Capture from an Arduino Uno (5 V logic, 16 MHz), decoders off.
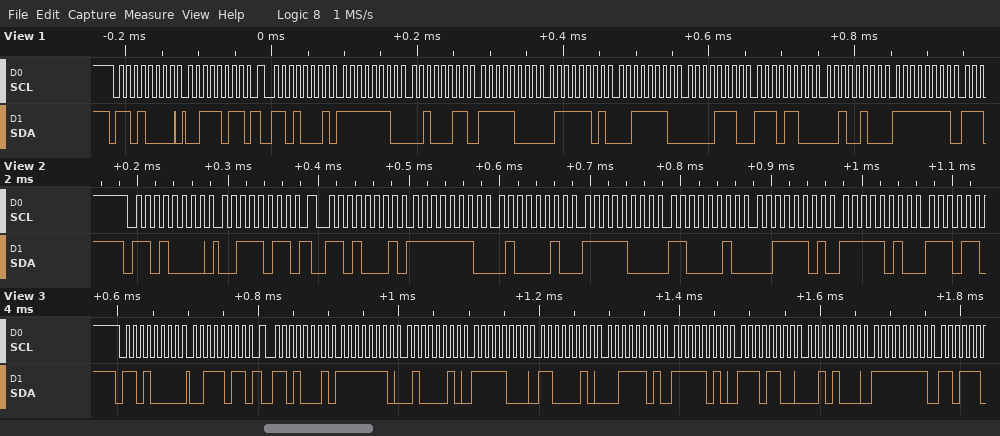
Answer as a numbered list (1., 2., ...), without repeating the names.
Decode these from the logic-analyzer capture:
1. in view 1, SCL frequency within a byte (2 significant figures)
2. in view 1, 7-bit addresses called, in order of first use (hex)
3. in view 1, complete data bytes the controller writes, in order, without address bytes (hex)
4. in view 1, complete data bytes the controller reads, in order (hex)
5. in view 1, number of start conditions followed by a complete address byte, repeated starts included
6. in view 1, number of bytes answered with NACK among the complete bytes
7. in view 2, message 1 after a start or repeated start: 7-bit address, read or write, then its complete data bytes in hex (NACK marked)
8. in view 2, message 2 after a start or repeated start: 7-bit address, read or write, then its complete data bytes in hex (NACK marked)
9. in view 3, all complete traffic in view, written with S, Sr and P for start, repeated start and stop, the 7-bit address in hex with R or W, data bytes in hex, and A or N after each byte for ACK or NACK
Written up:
1. 100 kHz
2. 0x68
3. 3B
4. FE 23 F8 7D 3E 0E EC 24 FF
5. 2
6. 0
7. 0x68 write: 3B
8. 0x68 read: FE 42 F8 C2 3D FA
9. S 68W A 3B A Sr 68R A FE A 42 A F8 A C2 A 3D A FA A EC A 28 A FF A
